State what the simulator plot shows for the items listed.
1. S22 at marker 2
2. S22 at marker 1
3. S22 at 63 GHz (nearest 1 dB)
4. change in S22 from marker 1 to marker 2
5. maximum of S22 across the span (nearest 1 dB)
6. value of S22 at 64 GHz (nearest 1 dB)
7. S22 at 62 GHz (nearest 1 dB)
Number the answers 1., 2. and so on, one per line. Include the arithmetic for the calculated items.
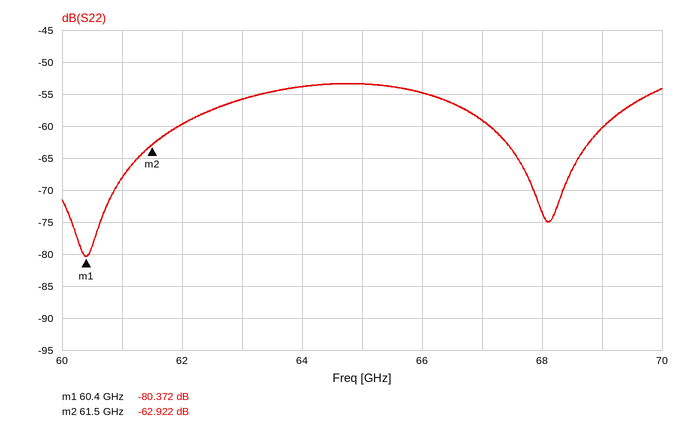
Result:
1. -62.922 dB
2. -80.372 dB
3. -56 dB
4. -62.922 − (-80.372) = 17.450 dB
5. -53 dB
6. -54 dB
7. -60 dB
